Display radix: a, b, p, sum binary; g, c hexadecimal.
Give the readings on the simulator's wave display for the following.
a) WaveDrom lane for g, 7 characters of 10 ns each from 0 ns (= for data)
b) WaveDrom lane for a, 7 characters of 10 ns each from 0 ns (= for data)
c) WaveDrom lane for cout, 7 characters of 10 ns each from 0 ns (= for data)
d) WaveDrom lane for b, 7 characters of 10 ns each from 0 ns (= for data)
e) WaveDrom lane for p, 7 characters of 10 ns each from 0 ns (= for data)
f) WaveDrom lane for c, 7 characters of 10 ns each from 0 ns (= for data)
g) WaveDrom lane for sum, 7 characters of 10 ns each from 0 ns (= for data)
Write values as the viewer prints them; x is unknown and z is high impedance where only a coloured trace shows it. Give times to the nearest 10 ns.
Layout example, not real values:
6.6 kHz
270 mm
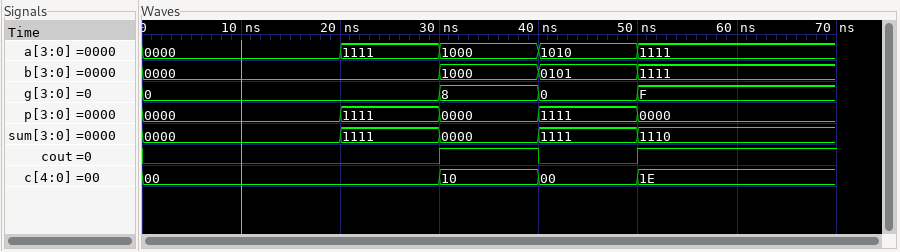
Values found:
{name: 'g', wave: '=..===.', data: '0 8 0 F'}
{name: 'a', wave: '=.====.', data: '0000 1111 1000 1010 1111'}
{name: 'cout', wave: '0..101.'}
{name: 'b', wave: '=..===.', data: '0000 1000 0101 1111'}
{name: 'p', wave: '=.====.', data: '0000 1111 0000 1111 0000'}
{name: 'c', wave: '=..===.', data: '00 10 00 1E'}
{name: 'sum', wave: '=.====.', data: '0000 1111 0000 1111 1110'}
